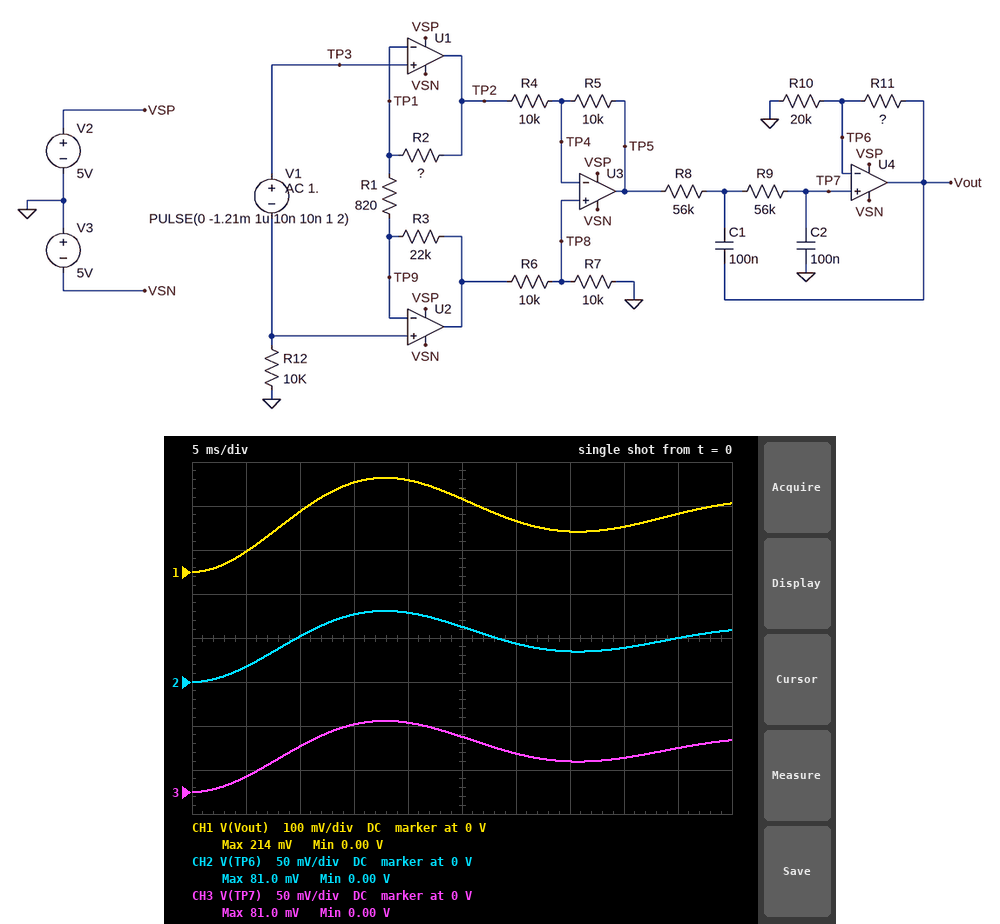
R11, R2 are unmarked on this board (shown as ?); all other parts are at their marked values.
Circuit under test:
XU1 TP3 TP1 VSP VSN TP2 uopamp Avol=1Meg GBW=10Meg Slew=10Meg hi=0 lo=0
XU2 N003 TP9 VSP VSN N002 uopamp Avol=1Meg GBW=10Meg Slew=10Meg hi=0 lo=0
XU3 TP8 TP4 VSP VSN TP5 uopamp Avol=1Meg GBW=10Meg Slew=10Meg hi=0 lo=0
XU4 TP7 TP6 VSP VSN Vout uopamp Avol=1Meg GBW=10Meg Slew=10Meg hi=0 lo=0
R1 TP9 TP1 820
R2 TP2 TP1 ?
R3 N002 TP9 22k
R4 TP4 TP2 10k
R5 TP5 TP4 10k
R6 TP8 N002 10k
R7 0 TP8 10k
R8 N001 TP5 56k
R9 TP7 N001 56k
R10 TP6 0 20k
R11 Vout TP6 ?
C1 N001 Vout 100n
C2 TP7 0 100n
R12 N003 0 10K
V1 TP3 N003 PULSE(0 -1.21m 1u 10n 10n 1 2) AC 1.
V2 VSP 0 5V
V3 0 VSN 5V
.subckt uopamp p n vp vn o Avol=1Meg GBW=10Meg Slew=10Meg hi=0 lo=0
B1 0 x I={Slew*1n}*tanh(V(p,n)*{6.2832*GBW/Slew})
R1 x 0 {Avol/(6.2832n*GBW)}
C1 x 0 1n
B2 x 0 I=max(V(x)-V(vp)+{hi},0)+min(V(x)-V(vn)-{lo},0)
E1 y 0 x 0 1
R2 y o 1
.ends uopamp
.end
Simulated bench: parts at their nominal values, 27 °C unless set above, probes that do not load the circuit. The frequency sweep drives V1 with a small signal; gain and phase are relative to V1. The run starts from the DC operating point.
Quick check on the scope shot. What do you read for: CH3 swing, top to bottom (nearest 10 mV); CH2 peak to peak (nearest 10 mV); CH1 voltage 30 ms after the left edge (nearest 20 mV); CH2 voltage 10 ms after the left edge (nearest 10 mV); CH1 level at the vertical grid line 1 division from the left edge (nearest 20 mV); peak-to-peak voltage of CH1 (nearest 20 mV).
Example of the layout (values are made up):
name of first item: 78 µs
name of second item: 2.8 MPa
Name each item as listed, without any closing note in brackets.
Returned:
CH3 swing, top to bottom: 80 mV
CH2 peak to peak: 80 mV
CH1 voltage 30 ms after the left edge: 120 mV
CH2 voltage 10 ms after the left edge: 50 mV
CH1 level at the vertical grid line 1 division from the left edge: 40 mV
peak-to-peak voltage of CH1: 220 mV
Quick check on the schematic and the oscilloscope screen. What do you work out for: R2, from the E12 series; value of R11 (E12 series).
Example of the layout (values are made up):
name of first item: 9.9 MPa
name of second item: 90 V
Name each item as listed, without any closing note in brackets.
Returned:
R2, from the E12 series: 12 kΩ
value of R11: 33 kΩ
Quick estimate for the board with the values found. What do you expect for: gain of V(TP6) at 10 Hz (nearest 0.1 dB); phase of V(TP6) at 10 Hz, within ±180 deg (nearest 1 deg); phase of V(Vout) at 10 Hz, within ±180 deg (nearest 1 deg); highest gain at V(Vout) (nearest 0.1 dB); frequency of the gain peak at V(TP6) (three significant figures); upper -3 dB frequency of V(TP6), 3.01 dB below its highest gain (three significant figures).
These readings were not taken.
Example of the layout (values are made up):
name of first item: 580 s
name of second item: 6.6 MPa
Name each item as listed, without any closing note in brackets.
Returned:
gain of V(TP6) at 10 Hz: 33.6 dB
phase of V(TP6) at 10 Hz, within ±180 deg: 172 deg
phase of V(Vout) at 10 Hz, within ±180 deg: 172 deg
highest gain at V(Vout): 50.3 dB
frequency of the gain peak at V(TP6): 27.5 Hz
upper -3 dB frequency of V(TP6), 3.01 dB below its highest gain: 32.2 Hz
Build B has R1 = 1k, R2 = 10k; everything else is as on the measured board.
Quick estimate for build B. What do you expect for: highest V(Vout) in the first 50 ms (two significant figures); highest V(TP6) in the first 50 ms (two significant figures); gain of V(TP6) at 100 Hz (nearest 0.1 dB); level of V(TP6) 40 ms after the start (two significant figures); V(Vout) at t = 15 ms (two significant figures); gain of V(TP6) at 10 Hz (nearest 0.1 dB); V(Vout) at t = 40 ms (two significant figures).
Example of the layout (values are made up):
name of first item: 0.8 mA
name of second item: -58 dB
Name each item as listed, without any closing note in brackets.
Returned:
highest V(Vout) in the first 50 ms: 170 mV
highest V(TP6) in the first 50 ms: 63 mV
gain of V(TP6) at 100 Hz: 9.2 dB
level of V(TP6) 40 ms after the start: 30 mV
V(Vout) at t = 15 ms: 160 mV
gain of V(TP6) at 10 Hz: 31.4 dB
V(Vout) at t = 40 ms: 80 mV
